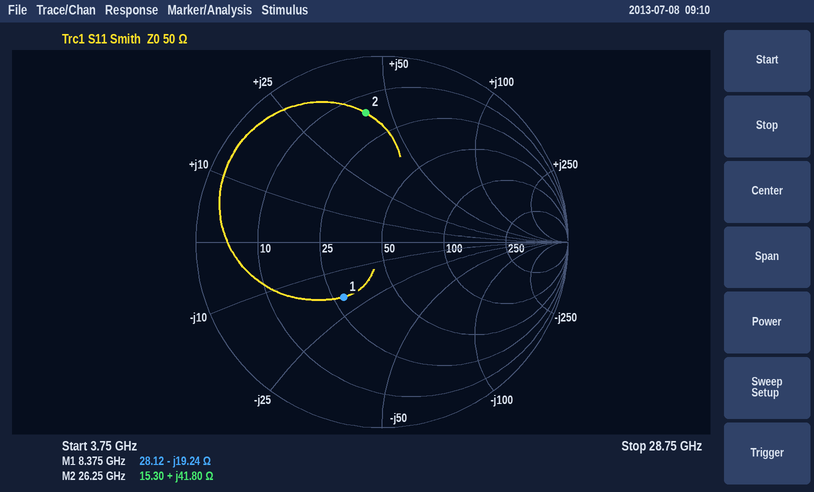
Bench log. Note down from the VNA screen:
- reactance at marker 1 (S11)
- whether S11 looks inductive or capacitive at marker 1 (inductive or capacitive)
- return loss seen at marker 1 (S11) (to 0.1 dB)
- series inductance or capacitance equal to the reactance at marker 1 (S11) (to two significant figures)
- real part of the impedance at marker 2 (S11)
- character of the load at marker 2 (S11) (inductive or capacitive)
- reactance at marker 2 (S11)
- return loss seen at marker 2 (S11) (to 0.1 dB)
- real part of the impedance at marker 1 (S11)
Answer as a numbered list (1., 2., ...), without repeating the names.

1. -19.24 Ω
2. capacitive
3. 8.8 dB
4. 990 fF
5. 15.30 Ω
6. inductive
7. +41.80 Ω
8. 3.1 dB
9. 28.12 Ω
